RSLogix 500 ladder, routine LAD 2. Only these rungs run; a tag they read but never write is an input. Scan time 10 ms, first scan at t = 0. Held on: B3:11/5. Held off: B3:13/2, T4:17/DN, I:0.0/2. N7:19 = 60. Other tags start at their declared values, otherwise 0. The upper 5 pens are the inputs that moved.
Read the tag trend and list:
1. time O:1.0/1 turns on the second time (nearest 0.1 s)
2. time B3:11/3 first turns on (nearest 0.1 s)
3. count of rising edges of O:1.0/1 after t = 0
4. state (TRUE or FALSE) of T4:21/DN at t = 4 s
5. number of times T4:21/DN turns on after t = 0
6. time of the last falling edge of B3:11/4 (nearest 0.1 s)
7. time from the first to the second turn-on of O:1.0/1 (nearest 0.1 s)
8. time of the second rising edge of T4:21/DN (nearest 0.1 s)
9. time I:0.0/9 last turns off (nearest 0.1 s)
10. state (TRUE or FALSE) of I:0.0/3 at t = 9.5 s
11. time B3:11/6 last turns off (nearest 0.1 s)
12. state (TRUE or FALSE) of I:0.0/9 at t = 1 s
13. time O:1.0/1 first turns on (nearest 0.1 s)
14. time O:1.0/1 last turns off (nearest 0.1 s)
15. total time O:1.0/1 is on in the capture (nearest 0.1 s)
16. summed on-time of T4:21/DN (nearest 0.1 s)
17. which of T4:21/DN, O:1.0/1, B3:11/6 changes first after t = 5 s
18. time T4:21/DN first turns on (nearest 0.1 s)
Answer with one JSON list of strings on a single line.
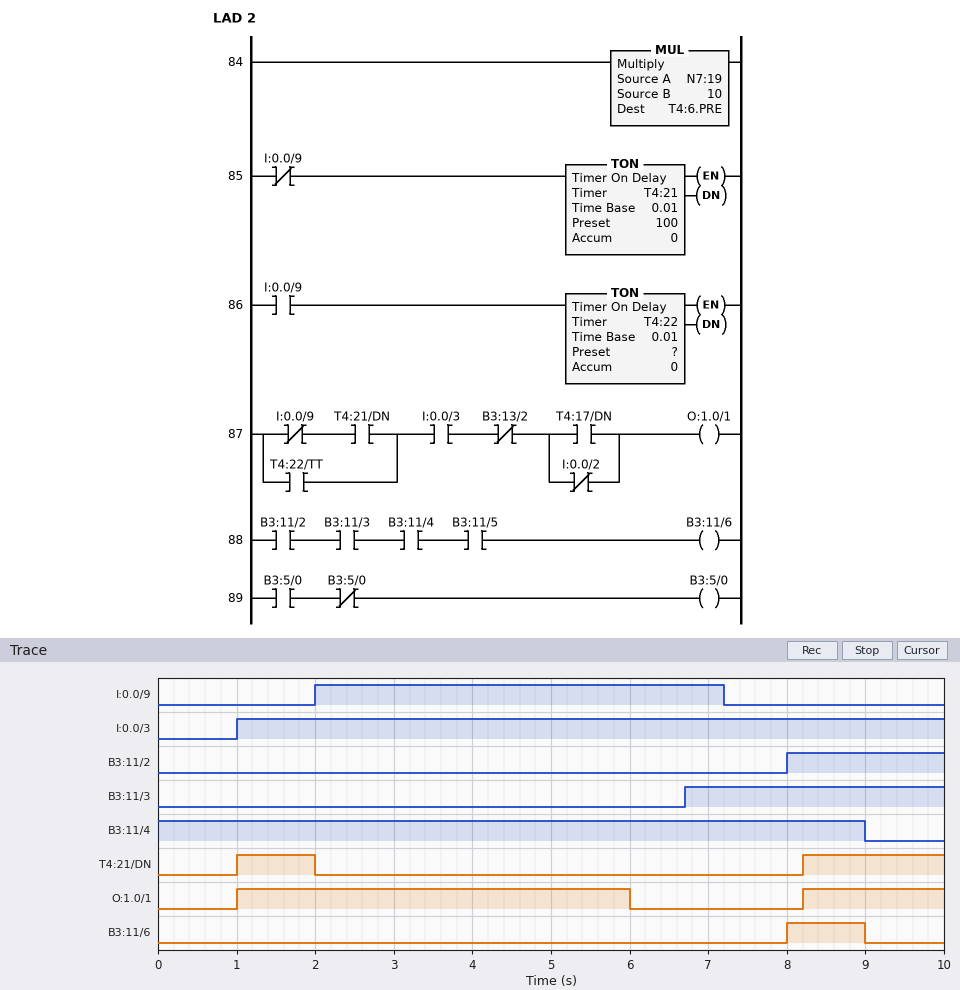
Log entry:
["8.2 s", "6.7 s", "2", "FALSE", "2", "9.0 s", "7.2 s", "8.2 s", "7.2 s", "TRUE", "9.0 s", "FALSE", "1.0 s", "6.0 s", "6.8 s", "2.8 s", "O:1.0/1", "1.0 s"]
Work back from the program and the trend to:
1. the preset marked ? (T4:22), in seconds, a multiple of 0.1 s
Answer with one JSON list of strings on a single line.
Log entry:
["4.0 s"]
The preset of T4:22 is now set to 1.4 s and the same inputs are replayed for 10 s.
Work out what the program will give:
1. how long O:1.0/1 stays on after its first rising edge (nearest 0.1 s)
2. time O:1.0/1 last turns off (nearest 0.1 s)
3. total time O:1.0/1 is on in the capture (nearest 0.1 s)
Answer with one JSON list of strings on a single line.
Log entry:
["2.4 s", "3.4 s", "4.2 s"]
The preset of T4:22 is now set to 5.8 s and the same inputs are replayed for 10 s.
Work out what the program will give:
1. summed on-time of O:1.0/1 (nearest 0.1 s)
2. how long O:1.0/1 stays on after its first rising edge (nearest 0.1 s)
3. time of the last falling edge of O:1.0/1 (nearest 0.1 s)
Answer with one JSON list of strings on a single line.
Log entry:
["8.0 s", "6.2 s", "7.2 s"]
